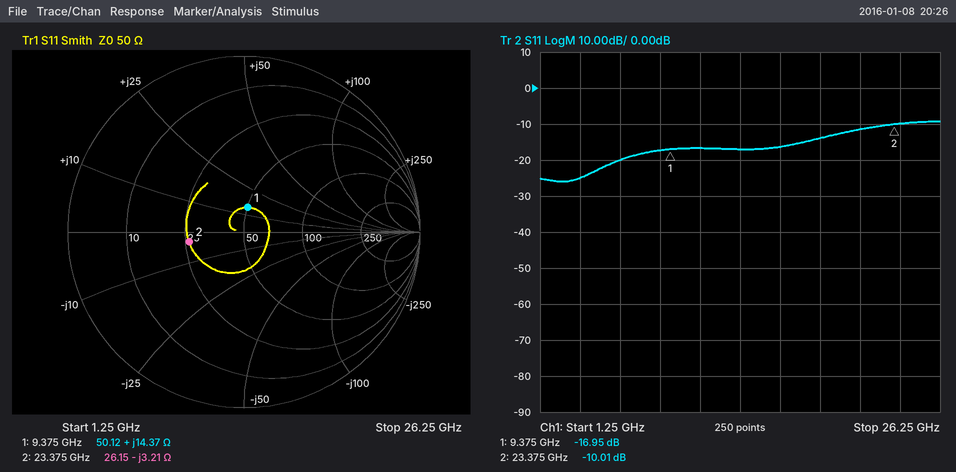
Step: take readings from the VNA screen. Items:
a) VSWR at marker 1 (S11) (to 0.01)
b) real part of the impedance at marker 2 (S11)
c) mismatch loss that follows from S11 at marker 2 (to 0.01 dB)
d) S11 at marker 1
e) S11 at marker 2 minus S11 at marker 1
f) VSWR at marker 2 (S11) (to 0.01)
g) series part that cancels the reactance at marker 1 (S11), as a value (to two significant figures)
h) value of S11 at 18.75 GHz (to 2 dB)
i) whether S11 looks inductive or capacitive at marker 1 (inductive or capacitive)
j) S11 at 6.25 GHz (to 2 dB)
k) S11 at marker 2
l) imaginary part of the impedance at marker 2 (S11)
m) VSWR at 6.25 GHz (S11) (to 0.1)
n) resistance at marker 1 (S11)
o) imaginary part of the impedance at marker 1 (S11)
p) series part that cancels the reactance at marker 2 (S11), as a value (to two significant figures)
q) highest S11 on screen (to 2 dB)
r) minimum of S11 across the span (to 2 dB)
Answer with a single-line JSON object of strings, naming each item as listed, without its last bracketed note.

{"VSWR at marker 1 (S11)": "1.33", "real part of the impedance at marker 2": "26.15 Ω", "mismatch loss that follows from S11 at marker 2": "0.46 dB", "S11 at marker 1": "-16.95 dB", "S11 at marker 2 minus S11 at marker 1": "6.94 dB", "VSWR at marker 2 (S11)": "1.92", "series part that cancels the reactance at marker 1 (S11), as a value": "1.2 pF", "value of S11 at 18.75 GHz": "-14 dB", "whether S11 looks inductive or capacitive at marker 1": "inductive", "S11 at 6.25 GHz": "-20 dB", "S11 at marker 2": "-10.01 dB", "imaginary part of the impedance at marker 2": "-3.21 Ω", "VSWR at 6.25 GHz (S11)": "1.2", "resistance at marker 1": "50.12 Ω", "imaginary part of the impedance at marker 1": "+14.37 Ω", "series part that cancels the reactance at marker 2 (S11), as a value": "22 pH", "highest S11 on screen": "-10 dB", "minimum of S11 across the span": "-26 dB"}
